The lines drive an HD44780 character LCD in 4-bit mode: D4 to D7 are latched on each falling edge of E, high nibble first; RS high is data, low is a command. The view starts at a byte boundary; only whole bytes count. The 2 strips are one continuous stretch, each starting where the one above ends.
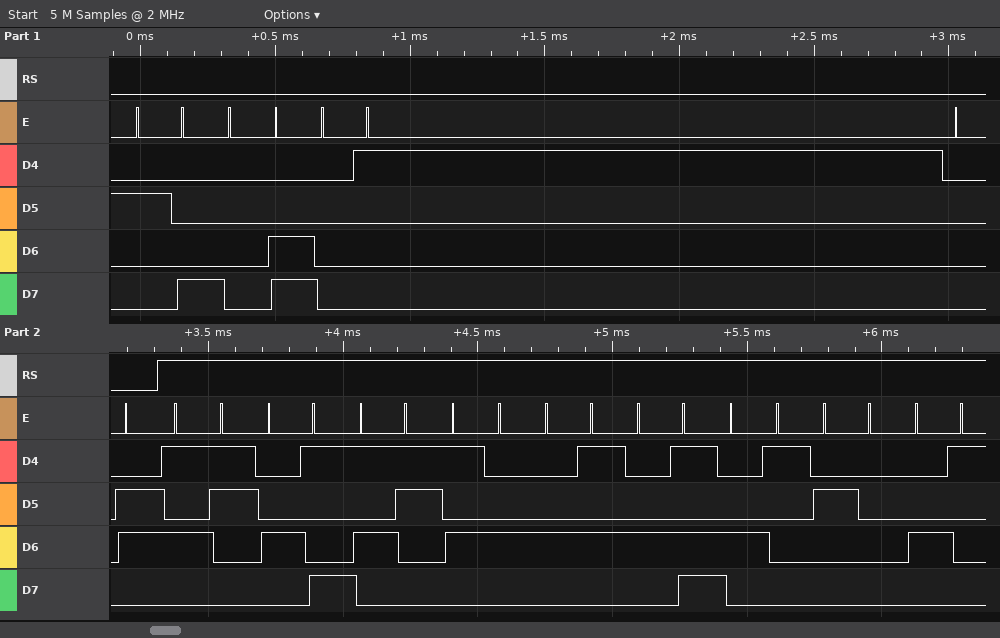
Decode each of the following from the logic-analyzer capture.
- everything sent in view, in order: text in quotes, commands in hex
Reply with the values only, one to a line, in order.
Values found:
0x28 0x0C 0x01 0x06 "SISTEMA A"
